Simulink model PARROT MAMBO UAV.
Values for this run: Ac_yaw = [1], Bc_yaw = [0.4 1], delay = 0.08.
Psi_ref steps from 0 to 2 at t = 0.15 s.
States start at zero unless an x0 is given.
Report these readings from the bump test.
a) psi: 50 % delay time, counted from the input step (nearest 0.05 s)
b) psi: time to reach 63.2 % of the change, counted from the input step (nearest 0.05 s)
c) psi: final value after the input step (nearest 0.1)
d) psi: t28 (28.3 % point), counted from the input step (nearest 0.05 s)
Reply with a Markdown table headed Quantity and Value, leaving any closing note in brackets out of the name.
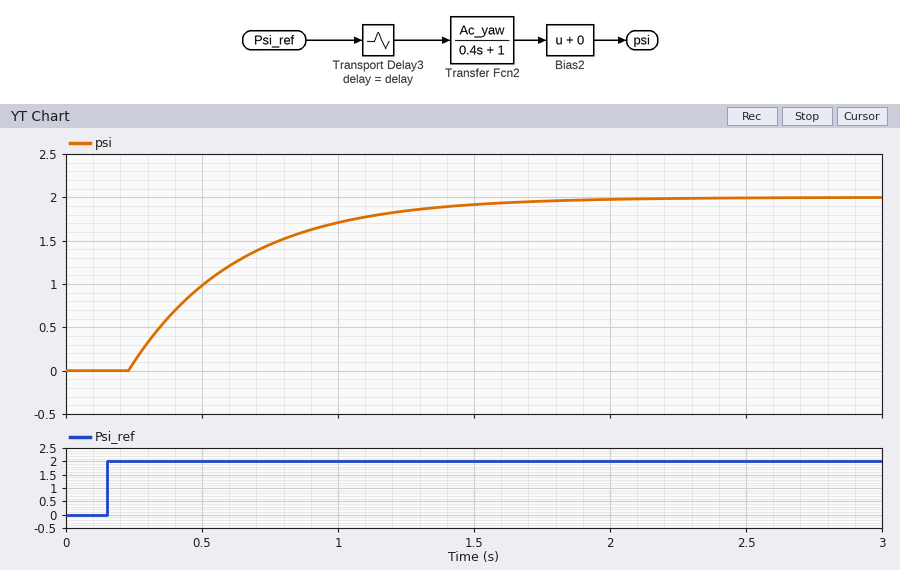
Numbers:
| Quantity | Value |
|---|---|
| psi: 50 % delay time, counted from the input step | 0.35 s |
| psi: time to reach 63.2 % of the change, counted from the input step | 0.50 s |
| psi: final value after the input step | 2.0 |
| psi: t28 (28.3 % point), counted from the input step | 0.20 s |
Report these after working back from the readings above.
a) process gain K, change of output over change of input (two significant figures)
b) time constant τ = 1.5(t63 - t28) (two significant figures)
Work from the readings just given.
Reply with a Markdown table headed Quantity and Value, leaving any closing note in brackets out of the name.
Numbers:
| Quantity | Value |
|---|---|
| process gain K, change of output over change of input | 1.0 |
| time constant τ = 1.5(t63 - t28) | 0.45 s |
